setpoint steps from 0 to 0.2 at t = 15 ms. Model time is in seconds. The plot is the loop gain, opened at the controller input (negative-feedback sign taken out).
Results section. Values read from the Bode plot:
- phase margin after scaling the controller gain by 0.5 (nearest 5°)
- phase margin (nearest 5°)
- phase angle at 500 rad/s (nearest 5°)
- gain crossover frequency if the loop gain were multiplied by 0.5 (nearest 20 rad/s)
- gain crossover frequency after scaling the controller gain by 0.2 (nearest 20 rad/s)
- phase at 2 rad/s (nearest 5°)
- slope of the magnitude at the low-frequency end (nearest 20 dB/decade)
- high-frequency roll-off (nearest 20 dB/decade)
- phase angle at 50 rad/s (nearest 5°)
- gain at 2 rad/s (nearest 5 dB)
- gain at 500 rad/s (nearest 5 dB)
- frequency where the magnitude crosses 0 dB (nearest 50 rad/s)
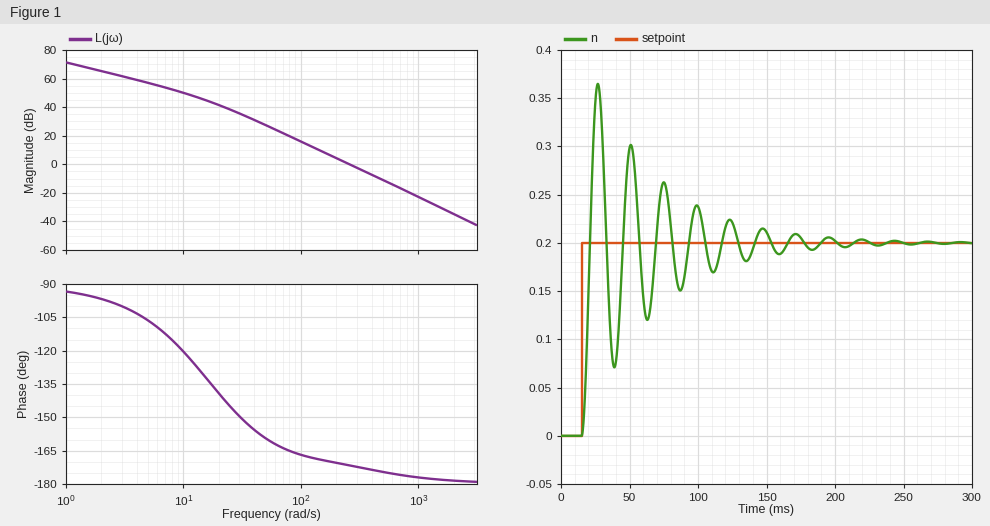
10°
10°
-175°
180 rad/s
120 rad/s
-95°
-20 dB/decade
-40 dB/decade
-160°
65 dB
-10 dB
250 rad/s
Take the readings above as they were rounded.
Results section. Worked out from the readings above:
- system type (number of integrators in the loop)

1
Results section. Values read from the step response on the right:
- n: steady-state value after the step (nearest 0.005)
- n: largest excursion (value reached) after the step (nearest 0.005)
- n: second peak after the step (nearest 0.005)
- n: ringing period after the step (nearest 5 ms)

0.200
0.365
0.300
25 ms
